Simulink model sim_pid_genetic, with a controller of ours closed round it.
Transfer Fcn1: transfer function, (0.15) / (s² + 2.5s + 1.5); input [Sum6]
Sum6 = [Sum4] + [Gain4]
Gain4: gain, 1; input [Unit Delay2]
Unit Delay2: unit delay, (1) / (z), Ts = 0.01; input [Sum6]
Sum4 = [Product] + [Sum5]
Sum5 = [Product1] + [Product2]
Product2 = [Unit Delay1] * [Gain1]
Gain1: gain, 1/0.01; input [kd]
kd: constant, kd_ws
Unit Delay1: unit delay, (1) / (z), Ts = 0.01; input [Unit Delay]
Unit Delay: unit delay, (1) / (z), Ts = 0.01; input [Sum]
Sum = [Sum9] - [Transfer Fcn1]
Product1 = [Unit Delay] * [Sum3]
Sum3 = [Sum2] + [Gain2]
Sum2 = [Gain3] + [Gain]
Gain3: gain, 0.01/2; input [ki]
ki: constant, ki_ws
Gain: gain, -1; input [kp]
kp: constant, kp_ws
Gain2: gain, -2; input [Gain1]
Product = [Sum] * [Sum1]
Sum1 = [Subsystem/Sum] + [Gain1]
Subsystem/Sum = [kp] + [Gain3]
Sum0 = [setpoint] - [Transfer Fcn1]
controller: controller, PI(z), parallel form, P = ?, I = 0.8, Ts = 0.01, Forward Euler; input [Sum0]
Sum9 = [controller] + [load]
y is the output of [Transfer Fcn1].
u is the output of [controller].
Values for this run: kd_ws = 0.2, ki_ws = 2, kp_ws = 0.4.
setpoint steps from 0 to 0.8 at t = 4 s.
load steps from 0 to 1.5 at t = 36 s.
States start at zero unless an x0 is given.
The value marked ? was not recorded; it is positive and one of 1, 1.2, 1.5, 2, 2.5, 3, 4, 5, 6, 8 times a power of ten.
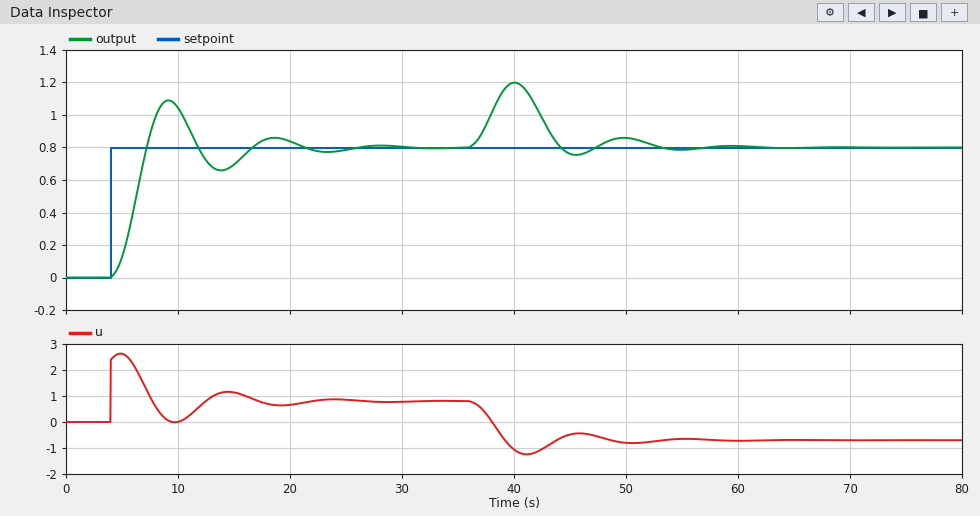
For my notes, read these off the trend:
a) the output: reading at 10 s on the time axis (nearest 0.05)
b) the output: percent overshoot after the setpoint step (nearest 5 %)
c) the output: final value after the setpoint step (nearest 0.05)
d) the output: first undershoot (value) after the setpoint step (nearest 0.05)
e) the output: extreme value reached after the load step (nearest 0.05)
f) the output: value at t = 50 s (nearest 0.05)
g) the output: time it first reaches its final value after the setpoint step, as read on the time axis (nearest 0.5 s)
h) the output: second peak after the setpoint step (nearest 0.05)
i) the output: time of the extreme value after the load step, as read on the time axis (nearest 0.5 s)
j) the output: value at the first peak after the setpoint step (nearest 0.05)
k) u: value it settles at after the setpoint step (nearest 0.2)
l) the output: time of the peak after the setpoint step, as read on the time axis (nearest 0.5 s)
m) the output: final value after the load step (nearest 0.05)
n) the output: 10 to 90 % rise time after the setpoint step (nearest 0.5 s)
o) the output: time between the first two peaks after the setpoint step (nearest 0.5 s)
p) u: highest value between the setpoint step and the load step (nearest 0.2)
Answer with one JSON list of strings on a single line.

["1.05", "35 %", "0.80", "0.65", "1.20", "0.85", "7.0 s", "0.85", "40.0 s", "1.10", "0.8", "9.0 s", "0.80", "2.0 s", "9.5 s", "2.6"]
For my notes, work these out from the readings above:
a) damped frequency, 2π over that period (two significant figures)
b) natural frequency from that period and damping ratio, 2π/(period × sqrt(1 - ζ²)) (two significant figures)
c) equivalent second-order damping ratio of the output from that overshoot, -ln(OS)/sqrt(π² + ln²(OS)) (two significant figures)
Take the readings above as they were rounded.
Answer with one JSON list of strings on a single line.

["0.66 rad/s", "0.70 rad/s", "0.32"]
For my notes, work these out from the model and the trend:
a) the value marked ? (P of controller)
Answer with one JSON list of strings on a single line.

["3"]
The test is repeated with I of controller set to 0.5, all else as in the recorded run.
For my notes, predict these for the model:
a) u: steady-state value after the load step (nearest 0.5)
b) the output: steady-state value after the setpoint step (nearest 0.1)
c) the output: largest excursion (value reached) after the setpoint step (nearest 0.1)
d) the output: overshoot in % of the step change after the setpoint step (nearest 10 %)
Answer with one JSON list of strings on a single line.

["-0.5", "0.8", "1.0", "20 %"]
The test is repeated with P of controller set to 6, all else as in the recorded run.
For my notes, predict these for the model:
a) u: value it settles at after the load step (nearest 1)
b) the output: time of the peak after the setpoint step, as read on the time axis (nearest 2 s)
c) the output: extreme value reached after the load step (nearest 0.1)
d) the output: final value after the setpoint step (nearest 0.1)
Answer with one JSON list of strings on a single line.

["-1", "8 s", "1.1", "0.8"]
